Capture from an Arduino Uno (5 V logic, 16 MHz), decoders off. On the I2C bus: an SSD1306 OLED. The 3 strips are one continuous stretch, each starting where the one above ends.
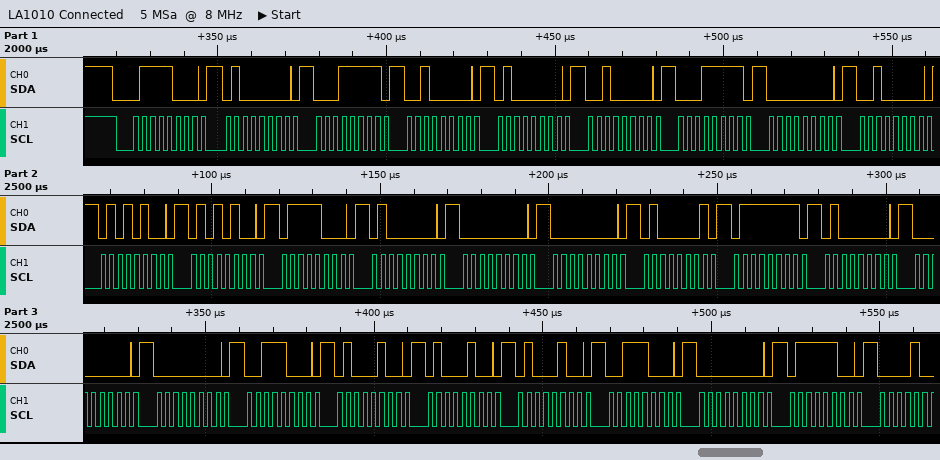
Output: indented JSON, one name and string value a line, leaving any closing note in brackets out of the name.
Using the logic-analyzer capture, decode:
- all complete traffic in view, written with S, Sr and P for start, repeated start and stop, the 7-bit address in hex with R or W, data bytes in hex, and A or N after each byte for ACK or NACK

{
  "all complete traffic in view, written with S, Sr and P for start, repeated start and stop, the 7-bit address in hex with R or W, data bytes in hex, and A or N after each byte for ACK or NACK": "S 3CW A 40 A 1F A 20 A 40 A 20 A 1F A 00 A 20 A 54 A 54 A 78 A 40 A 00 A 00 A 41 A 7F A 40 A 00 A 00 A 38 A 44 A 44 A 44 A 38 A 00 A 7C A"
}
